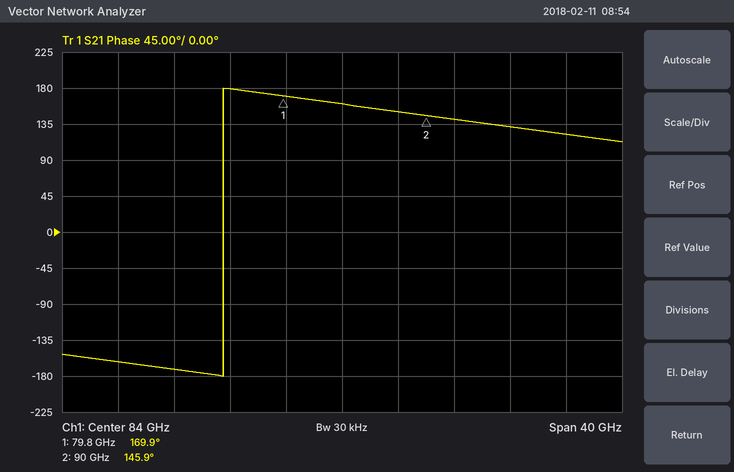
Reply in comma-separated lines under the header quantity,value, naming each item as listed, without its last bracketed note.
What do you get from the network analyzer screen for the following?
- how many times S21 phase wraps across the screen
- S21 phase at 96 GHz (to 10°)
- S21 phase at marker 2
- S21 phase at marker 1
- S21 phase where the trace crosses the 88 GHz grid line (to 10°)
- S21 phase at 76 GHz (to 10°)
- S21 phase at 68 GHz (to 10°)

quantity,value
how many times S21 phase wraps across the screen,1
S21 phase at 96 GHz,130°
S21 phase at marker 2,145.9°
S21 phase at marker 1,169.9°
S21 phase where the trace crosses the 88 GHz grid line,150°
S21 phase at 76 GHz,180°
S21 phase at 68 GHz,-160°
